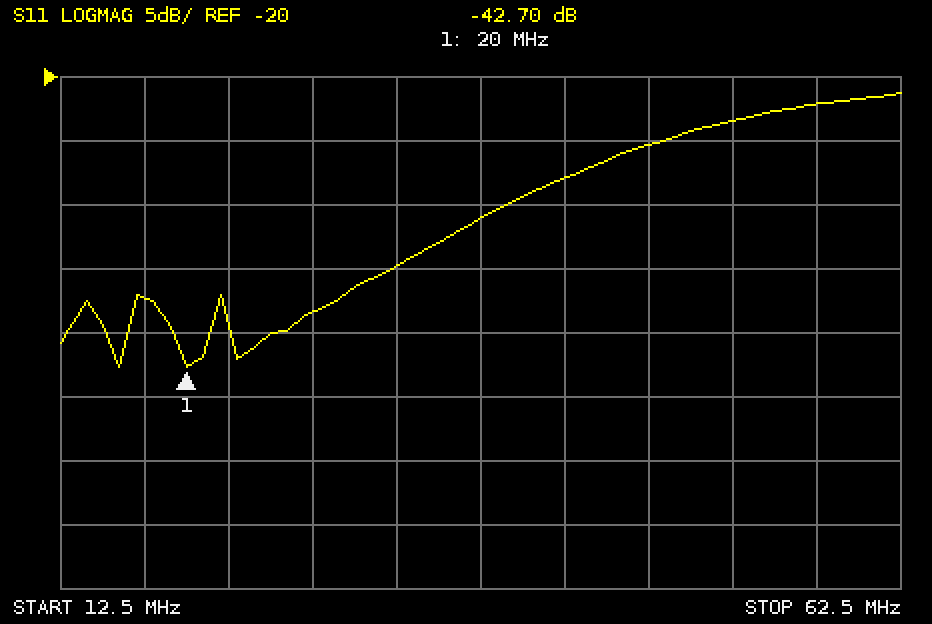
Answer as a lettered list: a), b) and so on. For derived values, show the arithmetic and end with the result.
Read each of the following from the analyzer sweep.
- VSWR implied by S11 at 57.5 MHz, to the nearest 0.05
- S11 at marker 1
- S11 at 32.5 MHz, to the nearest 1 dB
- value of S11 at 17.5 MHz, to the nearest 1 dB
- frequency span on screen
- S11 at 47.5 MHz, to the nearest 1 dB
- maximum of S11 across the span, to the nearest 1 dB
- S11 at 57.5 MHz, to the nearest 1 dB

a) |Γ| = 10^(-22/20) = 0.0794; VSWR = (1 + 0.0794)/(1 − 0.0794) ≈ 1.17, so 1.15 to the nearest 0.05
b) -42.70 dB
c) -35 dB
d) -37 dB
e) 50 MHz
f) -25 dB
g) -21 dB
h) -22 dB
